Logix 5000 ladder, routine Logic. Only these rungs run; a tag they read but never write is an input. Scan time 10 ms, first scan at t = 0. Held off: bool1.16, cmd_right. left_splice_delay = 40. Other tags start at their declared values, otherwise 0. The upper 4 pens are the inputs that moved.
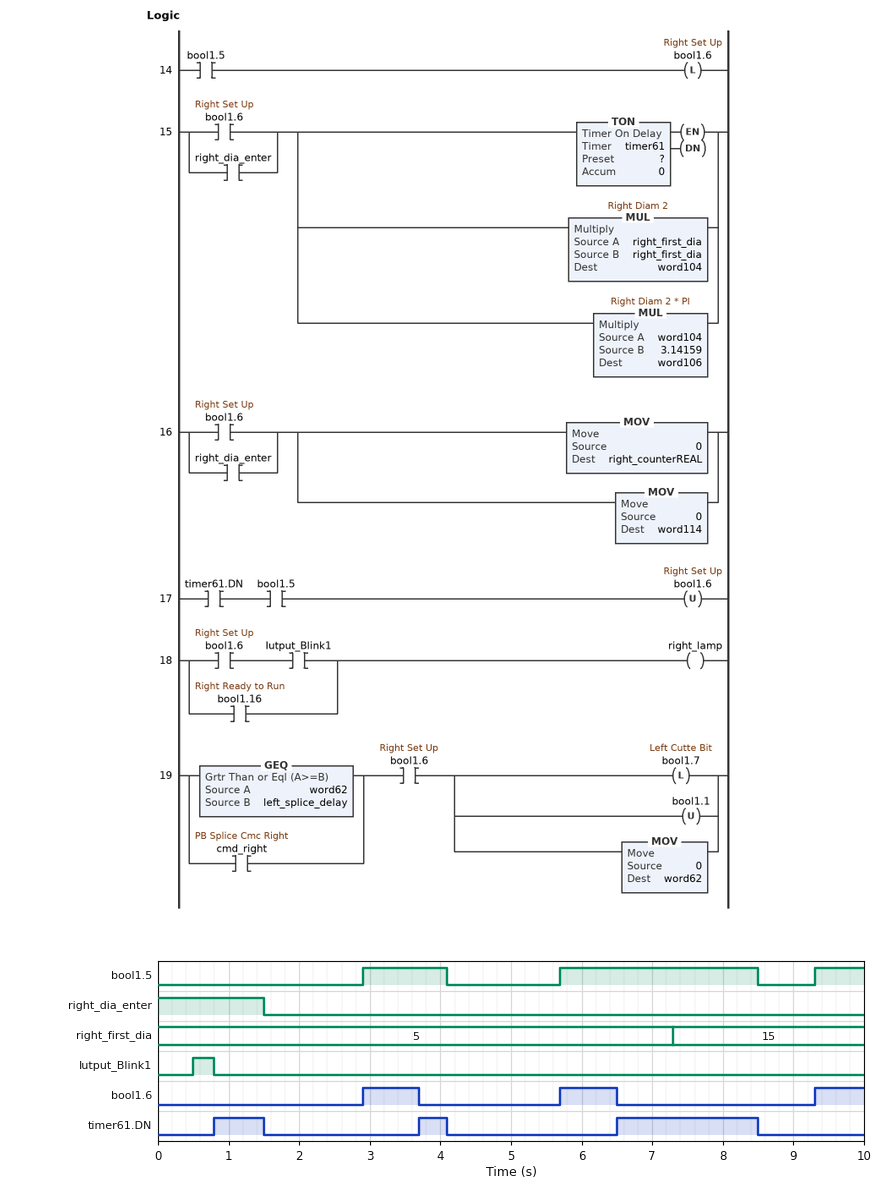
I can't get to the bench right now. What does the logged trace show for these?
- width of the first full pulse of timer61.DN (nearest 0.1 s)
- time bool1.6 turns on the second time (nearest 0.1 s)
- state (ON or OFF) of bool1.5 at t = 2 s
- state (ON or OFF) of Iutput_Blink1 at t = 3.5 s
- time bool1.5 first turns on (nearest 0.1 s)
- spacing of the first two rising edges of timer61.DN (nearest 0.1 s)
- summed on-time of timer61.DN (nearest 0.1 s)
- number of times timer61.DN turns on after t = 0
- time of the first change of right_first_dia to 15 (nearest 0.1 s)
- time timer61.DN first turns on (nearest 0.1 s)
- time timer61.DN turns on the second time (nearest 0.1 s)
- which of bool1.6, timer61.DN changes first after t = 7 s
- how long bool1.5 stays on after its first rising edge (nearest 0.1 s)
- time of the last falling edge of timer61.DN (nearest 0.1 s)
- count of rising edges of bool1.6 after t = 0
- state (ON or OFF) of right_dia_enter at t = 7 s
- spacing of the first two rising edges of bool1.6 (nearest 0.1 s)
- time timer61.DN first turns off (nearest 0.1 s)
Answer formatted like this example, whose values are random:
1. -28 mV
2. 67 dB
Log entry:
1. 0.7 s
2. 5.7 s
3. OFF
4. OFF
5. 2.9 s
6. 2.9 s
7. 3.1 s
8. 3
9. 7.3 s
10. 0.8 s
11. 3.7 s
12. timer61.DN
13. 1.2 s
14. 8.5 s
15. 3
16. OFF
17. 2.8 s
18. 1.5 s
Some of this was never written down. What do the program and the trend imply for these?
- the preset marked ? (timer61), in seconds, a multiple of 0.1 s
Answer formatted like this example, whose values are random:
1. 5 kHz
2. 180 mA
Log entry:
1. 0.8 s
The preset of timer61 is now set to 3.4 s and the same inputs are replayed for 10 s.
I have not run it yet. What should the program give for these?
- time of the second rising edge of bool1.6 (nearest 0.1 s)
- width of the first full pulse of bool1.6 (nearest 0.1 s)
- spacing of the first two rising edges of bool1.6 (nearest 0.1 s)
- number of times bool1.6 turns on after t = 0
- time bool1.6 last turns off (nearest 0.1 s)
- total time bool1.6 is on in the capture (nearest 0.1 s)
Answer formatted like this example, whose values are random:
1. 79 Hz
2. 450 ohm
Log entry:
1. 9.3 s
2. 3.4 s
3. 6.4 s
4. 2
5. 6.3 s
6. 4.1 s
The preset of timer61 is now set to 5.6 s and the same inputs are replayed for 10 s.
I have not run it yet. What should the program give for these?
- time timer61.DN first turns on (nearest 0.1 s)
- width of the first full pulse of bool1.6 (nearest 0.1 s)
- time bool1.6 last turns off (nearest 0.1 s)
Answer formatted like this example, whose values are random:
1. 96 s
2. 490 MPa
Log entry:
1. 8.5 s
2. 6.4 s
3. 9.3 s
